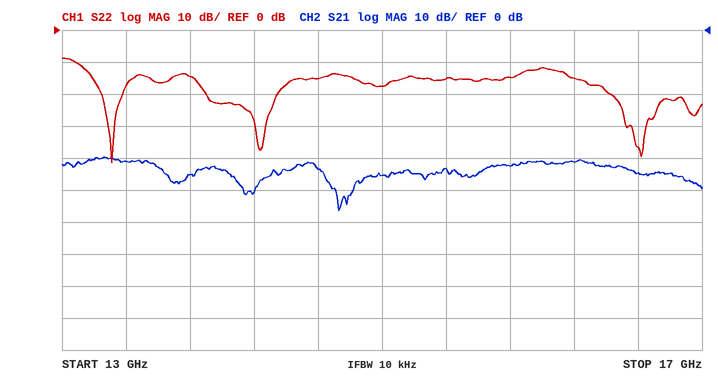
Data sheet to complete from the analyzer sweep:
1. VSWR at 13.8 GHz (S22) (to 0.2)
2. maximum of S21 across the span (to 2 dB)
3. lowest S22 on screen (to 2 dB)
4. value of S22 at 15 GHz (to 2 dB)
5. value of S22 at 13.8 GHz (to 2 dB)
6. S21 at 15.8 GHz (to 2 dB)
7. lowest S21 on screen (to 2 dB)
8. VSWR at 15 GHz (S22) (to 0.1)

1.4
-40 dB
-42 dB
-18 dB
-14 dB
-42 dB
-56 dB
1.3
